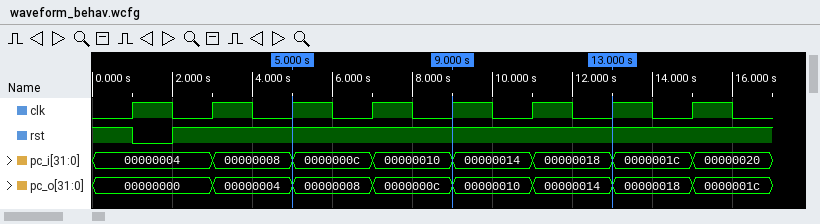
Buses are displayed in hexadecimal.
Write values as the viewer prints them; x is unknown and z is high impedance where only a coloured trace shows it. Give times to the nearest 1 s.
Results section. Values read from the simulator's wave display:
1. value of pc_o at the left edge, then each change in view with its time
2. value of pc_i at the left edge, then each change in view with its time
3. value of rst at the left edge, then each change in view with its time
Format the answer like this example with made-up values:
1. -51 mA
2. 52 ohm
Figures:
1. 00000000, 00000004 at 3 s, 00000008 at 5 s, 0000000c at 7 s, 00000010 at 9 s, 00000014 at 11 s, 00000018 at 13 s, 0000001c at 15 s
2. 00000004, 00000008 at 3 s, 0000000c at 5 s, 00000010 at 7 s, 00000014 at 9 s, 00000018 at 11 s, 0000001c at 13 s, 00000020 at 15 s
3. 1, 0 at 1 s, 1 at 2 s
